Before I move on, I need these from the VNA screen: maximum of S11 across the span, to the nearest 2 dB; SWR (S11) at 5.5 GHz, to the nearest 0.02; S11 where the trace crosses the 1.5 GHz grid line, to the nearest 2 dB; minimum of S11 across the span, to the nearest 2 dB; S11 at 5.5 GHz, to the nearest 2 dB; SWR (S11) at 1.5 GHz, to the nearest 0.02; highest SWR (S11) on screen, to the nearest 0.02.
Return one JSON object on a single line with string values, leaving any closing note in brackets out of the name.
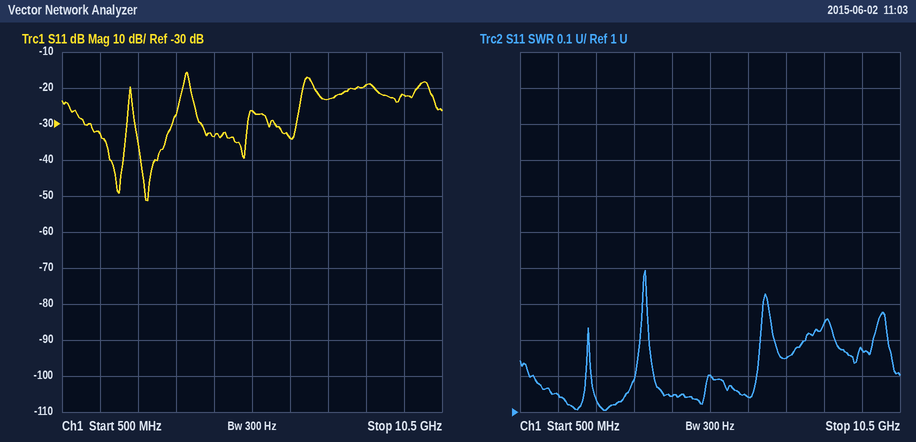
{"maximum of S11 across the span, to the nearest 2 dB": "-16 dB", "SWR (S11) at 5.5 GHz, to the nearest 0.02": "1.10", "S11 where the trace crosses the 1.5 GHz grid line, to the nearest 2 dB": "-32 dB", "minimum of S11 across the span, to the nearest 2 dB": "-52 dB", "S11 at 5.5 GHz, to the nearest 2 dB": "-26 dB", "SWR (S11) at 1.5 GHz, to the nearest 0.02": "1.04", "highest SWR (S11) on screen, to the nearest 0.02": "1.40"}
